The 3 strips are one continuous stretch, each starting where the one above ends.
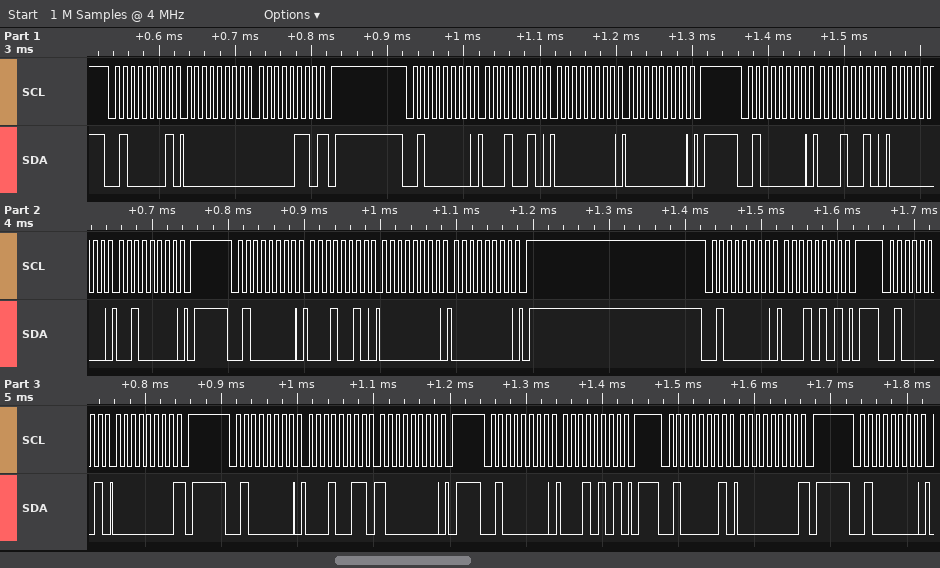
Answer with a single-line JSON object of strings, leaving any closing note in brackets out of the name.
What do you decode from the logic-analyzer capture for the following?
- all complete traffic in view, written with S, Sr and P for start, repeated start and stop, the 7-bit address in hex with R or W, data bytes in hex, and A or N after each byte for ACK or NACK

{"all complete traffic in view, written with S, Sr and P for start, repeated start and stop, the 7-bit address in hex with R or W, data bytes in hex, and A or N after each byte for ACK or NACK": "S 20R A 00 A 06 N P S 20W A 12 A 00 A 00 A P S 20W A 12 A 00 A 20 A P S 20W A 12 A 00 A 00 A P S 20W A 15 A P S 20R A 00 N P S 20W A 13 A 80 A P S 20W A 15 A P S 20R A 00 N P S 20W A"}
